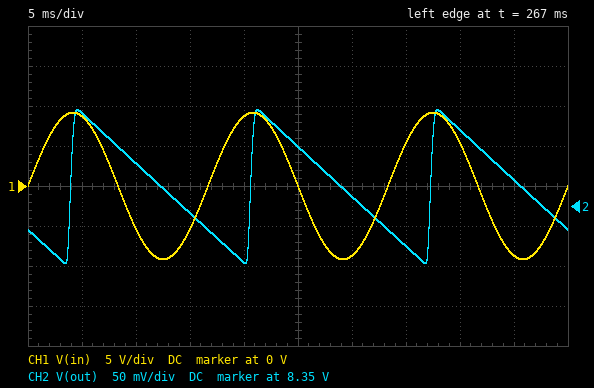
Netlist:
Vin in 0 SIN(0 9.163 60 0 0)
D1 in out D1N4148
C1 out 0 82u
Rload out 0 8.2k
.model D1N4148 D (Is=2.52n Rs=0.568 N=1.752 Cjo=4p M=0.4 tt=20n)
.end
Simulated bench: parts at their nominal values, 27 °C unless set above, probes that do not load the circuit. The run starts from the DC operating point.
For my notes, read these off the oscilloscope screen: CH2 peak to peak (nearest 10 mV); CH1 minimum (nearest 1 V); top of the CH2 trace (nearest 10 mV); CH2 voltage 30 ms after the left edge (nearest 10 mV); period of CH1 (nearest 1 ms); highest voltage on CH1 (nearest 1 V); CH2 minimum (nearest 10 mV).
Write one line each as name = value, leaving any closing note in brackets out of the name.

CH2 peak to peak = 190 mV
CH1 minimum = -9 V
top of the CH2 trace = 8.47 V
CH2 voltage 30 ms after the left edge = 8.36 V
period of CH1 = 17 ms
highest voltage on CH1 = 9 V
CH2 minimum = 8.28 V
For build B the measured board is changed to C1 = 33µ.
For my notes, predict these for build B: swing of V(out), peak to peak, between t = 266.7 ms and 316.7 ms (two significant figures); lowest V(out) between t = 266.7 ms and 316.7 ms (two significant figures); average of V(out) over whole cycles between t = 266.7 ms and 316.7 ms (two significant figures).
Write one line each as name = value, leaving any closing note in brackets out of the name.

swing of V(out), peak to peak, between t = 266.7 ms and 316.7 ms = 470 mV
lowest V(out) between t = 266.7 ms and 316.7 ms = 8.0 V
average of V(out) over whole cycles between t = 266.7 ms and 316.7 ms = 8.3 V
